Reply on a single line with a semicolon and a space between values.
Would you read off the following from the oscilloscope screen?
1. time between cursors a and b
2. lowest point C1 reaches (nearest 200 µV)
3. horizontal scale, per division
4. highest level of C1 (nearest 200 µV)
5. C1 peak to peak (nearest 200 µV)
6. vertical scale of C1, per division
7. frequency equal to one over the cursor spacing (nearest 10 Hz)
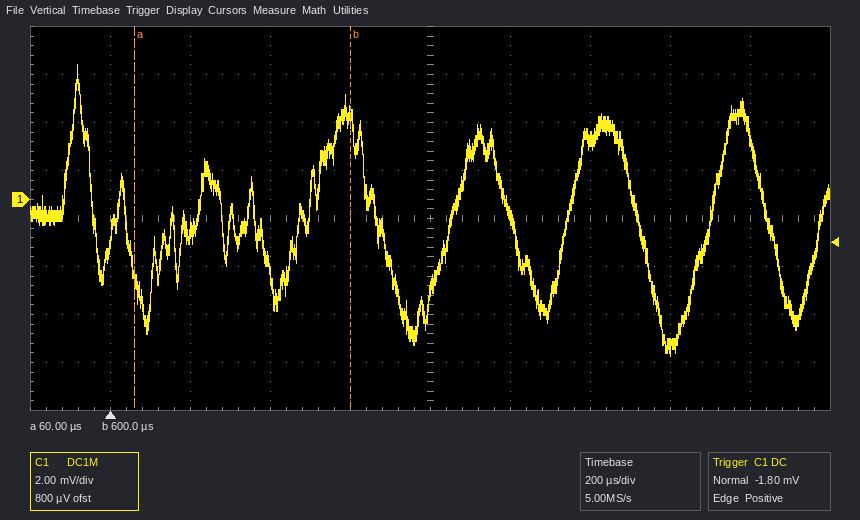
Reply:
540 µs; -6.6 mV; 200 µs; 5.6 mV; 12.2 mV; 2 mV; 1.85 kHz
